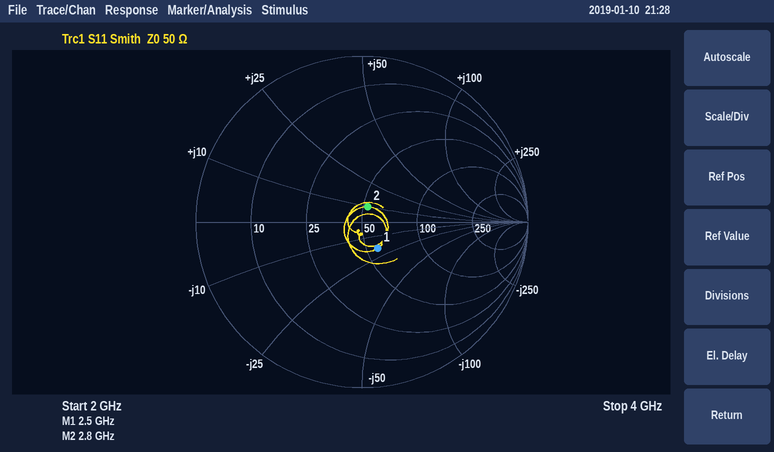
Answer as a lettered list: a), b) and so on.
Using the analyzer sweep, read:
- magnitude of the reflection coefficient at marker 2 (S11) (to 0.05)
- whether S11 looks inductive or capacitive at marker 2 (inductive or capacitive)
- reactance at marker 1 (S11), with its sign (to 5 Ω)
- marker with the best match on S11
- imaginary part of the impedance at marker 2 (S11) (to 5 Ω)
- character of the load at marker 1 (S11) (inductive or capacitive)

a) 0.10
b) inductive
c) -20 Ω
d) marker 2
e) +10 Ω
f) capacitive
